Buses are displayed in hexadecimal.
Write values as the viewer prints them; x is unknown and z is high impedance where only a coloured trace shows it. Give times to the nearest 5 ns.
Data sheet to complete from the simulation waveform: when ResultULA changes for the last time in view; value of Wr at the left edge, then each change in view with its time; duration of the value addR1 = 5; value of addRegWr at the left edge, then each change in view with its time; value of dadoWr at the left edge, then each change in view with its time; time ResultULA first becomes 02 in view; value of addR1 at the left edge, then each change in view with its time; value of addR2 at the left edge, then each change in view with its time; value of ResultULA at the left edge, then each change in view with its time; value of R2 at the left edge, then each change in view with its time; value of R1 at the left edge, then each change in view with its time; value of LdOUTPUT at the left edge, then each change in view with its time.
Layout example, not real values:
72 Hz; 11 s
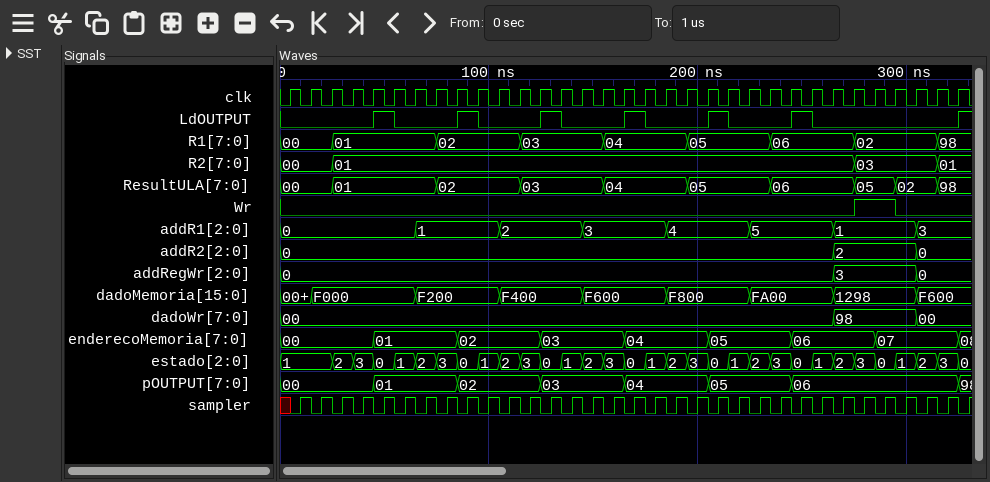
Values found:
315 ns; 0, 1 at 275 ns, 0 at 295 ns; 40 ns; 0, 3 at 265 ns, 0 at 305 ns; 00, 98 at 265 ns, 00 at 305 ns; 75 ns; 0, 1 at 65 ns, 2 at 105 ns, 3 at 145 ns, 4 at 185 ns, 5 at 225 ns, 1 at 265 ns, 3 at 305 ns; 0, 2 at 265 ns, 0 at 305 ns; 00, 01 at 25 ns, 02 at 75 ns, 03 at 115 ns, 04 at 155 ns, 05 at 195 ns, 06 at 235 ns, 05 at 275 ns, 02 at 295 ns, 98 at 315 ns; 00, 01 at 25 ns, 03 at 275 ns, 01 at 315 ns; 00, 01 at 25 ns, 02 at 75 ns, 03 at 115 ns, 04 at 155 ns, 05 at 195 ns, 06 at 235 ns, 02 at 275 ns, 98 at 315 ns; 0, 1 at 45 ns, 0 at 55 ns, 1 at 85 ns, 0 at 95 ns, 1 at 125 ns, 0 at 135 ns, 1 at 165 ns, 0 at 175 ns, 1 at 205 ns, 0 at 215 ns, 1 at 245 ns, 0 at 255 ns, 1 at 325 ns
